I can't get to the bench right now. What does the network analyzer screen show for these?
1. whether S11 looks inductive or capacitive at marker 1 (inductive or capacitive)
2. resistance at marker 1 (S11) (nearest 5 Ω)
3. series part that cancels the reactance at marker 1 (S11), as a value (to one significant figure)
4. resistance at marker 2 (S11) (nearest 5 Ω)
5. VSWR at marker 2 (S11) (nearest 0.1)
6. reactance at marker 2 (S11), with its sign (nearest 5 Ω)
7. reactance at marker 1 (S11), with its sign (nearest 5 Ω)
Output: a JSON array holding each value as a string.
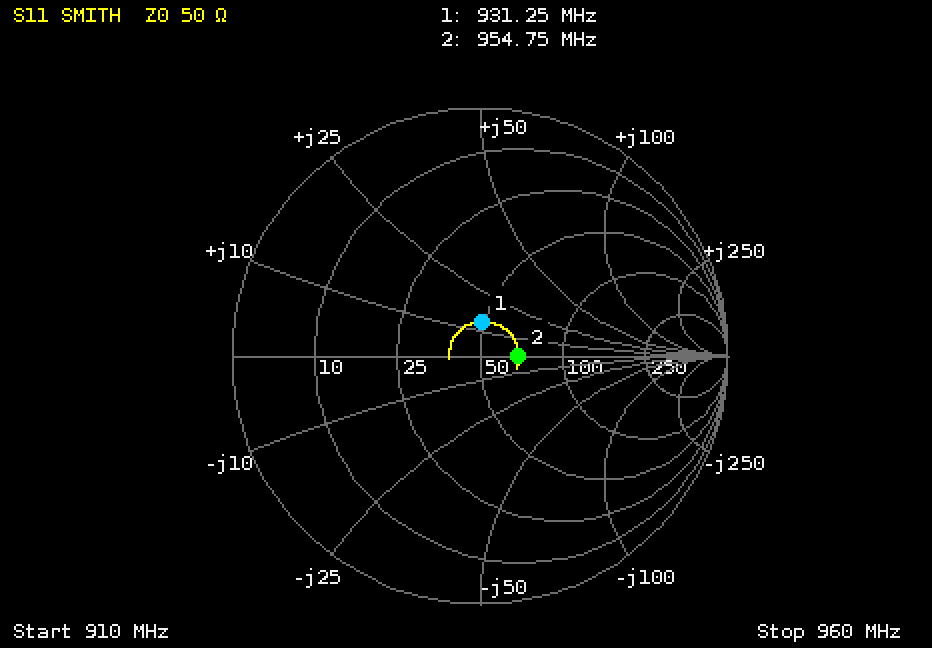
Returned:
["inductive", "50 Ω", "10 pF", "70 Ω", "1.4", "0 Ω", "+15 Ω"]
